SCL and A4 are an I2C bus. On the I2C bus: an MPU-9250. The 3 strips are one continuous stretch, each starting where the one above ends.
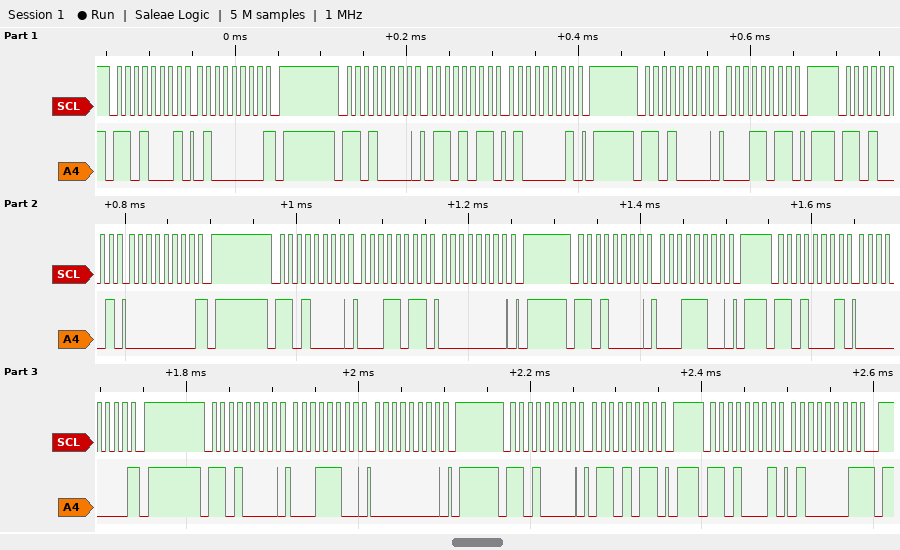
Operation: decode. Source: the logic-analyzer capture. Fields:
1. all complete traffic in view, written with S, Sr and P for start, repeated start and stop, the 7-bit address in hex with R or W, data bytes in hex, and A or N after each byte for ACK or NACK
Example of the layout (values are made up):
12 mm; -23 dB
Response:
S 68R A 40 N P S 68W A 6B A 41 A P S 68W A 1B A P S 68R A 00 N P S 68W A 1B A 00 A P S 68W A 1C A P S 68R A 00 N P S 68W A 1C A 00 A P S 68W A 6B A P S 68R A 41 N P
